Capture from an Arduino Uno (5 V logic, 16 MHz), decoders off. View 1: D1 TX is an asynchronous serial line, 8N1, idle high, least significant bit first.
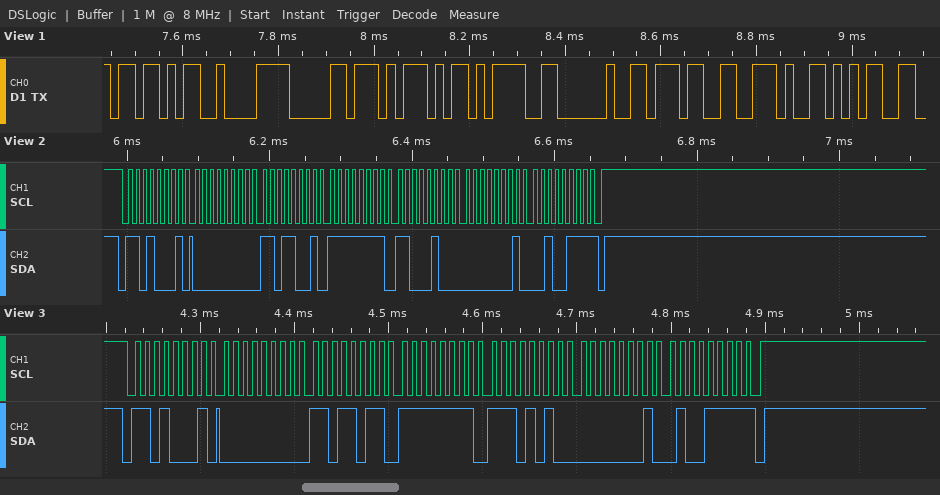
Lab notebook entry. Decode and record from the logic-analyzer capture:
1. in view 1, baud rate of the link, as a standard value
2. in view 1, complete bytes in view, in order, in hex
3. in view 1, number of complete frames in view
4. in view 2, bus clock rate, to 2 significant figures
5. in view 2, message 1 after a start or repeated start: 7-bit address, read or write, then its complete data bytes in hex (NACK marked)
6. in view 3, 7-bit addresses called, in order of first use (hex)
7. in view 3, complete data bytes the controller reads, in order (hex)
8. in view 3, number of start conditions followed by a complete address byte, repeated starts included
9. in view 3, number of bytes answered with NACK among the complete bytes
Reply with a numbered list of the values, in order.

1. 57600 baud
2. 0x5B 0xC2 0xB0 0x5D 0x3D 0x20 0x37 0x2E 0x35
3. 9
4. 100 kHz
5. 0x68 read: 00 D9 FF C4 01 27 NACK
6. 0x68
7. 00 DB FF EA 01 4F
8. 1
9. 1
